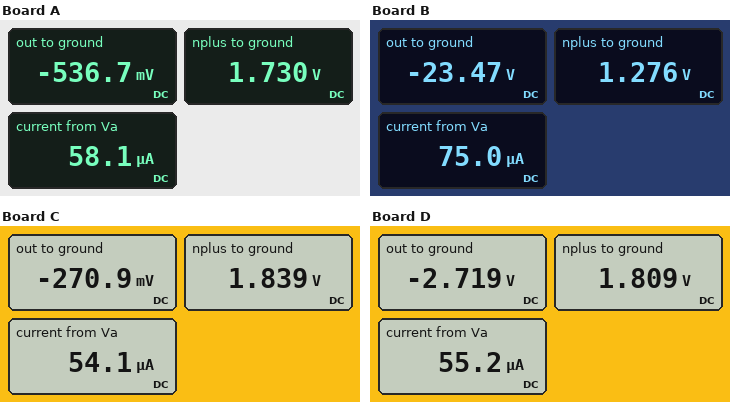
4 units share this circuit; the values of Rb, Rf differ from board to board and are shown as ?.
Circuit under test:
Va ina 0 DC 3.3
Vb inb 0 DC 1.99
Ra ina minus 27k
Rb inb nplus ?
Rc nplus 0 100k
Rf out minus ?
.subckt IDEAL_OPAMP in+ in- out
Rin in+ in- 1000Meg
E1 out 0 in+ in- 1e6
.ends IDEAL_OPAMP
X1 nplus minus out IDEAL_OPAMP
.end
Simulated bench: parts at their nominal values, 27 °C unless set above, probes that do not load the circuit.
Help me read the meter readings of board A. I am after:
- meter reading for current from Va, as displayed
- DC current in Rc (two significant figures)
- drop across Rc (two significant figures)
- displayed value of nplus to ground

58.1 µA
17 µA
1.7 V
1.730 V
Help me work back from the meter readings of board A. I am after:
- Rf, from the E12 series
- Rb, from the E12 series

39 kΩ
15 kΩ
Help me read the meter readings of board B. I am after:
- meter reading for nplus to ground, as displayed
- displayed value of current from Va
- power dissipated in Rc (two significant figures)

1.276 V
75.0 µA
16 µW
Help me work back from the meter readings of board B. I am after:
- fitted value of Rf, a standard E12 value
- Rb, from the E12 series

330 kΩ
56 kΩ
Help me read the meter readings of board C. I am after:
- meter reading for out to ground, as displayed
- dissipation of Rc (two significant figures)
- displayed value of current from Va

-270.9 mV
34 µW
54.1 µA
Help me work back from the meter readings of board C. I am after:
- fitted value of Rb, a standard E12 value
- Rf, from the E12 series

8.2 kΩ
39 kΩ
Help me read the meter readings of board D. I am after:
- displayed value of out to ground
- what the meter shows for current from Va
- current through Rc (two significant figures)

-2.719 V
55.2 µA
18 µA
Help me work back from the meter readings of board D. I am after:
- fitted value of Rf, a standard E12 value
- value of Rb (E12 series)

82 kΩ
10 kΩ
